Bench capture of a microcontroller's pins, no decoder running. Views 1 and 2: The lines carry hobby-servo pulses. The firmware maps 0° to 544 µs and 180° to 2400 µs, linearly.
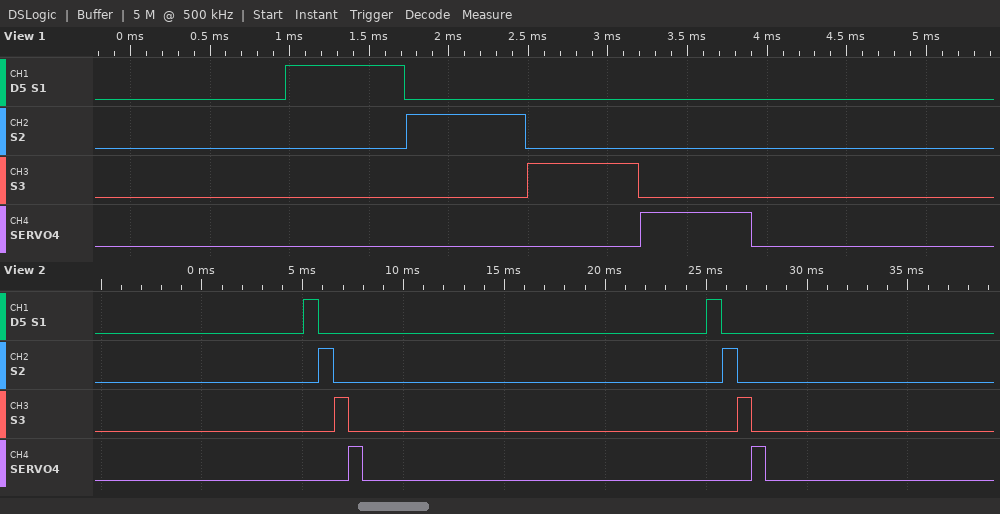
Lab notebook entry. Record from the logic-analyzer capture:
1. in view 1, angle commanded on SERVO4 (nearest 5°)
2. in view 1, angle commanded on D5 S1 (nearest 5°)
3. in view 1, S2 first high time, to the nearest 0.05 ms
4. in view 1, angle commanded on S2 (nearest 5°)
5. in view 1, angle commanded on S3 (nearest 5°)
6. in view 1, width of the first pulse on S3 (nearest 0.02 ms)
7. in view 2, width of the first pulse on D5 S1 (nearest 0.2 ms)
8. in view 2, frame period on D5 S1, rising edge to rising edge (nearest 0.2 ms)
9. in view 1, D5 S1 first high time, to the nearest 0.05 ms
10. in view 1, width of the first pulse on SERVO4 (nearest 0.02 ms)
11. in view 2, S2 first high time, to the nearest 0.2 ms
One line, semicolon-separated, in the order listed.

15°; 20°; 0.75 ms; 20°; 15°; 0.70 ms; 0.8 ms; 20.0 ms; 0.75 ms; 0.70 ms; 0.8 ms
